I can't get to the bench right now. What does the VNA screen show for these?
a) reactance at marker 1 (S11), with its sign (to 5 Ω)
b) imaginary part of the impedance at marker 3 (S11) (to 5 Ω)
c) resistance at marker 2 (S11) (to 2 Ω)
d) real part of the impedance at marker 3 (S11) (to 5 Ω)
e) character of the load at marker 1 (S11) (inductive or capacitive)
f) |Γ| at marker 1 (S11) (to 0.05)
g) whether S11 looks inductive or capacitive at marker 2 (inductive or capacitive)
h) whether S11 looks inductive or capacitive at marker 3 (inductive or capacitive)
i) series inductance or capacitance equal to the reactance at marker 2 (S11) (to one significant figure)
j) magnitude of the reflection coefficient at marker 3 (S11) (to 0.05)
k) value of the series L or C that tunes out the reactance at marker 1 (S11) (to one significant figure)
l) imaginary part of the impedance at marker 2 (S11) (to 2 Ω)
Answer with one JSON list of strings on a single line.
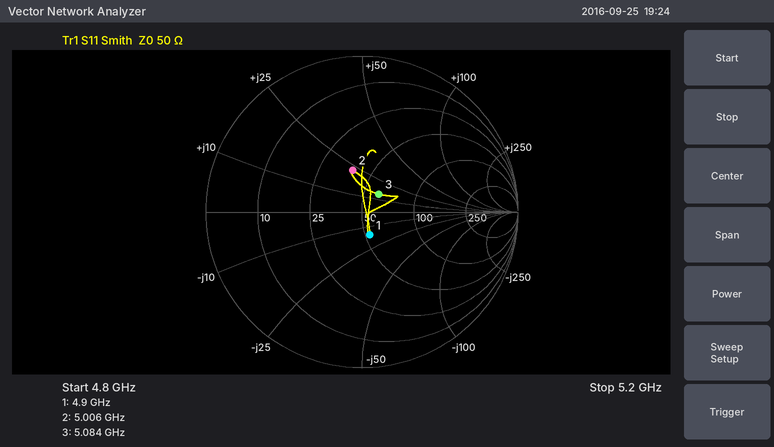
["-15 Ω", "+15 Ω", "38 Ω", "60 Ω", "capacitive", "0.15", "inductive", "inductive", "700 pH", "0.15", "500 pH", "+22 Ω"]
